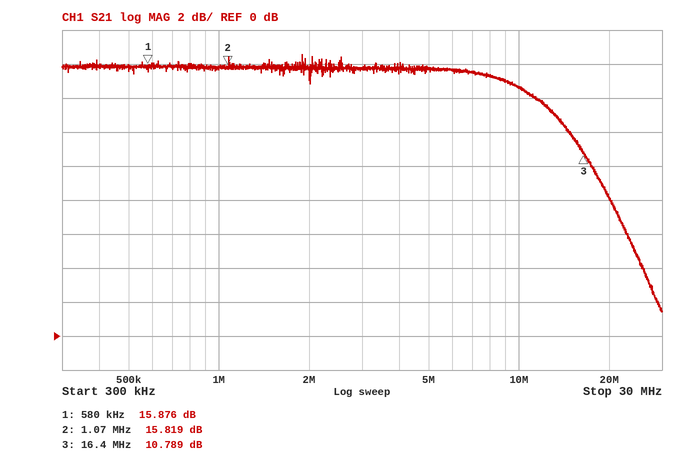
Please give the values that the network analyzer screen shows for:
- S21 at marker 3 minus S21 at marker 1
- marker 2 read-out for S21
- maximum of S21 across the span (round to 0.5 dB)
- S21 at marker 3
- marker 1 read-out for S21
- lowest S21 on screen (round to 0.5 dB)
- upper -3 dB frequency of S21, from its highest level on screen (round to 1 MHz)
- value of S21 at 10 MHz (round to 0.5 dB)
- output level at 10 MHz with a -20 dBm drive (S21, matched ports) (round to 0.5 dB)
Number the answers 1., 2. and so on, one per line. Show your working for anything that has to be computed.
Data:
1. 10.789 − (15.876) = -5.087 dB
2. 15.819 dB
3. 16.5 dB
4. 10.789 dB
5. 15.876 dB
6. 1.5 dB
7. 12 MHz
8. 14.5 dB
9. -20 dBm + (14.5 dB) = -5.5 dBm
